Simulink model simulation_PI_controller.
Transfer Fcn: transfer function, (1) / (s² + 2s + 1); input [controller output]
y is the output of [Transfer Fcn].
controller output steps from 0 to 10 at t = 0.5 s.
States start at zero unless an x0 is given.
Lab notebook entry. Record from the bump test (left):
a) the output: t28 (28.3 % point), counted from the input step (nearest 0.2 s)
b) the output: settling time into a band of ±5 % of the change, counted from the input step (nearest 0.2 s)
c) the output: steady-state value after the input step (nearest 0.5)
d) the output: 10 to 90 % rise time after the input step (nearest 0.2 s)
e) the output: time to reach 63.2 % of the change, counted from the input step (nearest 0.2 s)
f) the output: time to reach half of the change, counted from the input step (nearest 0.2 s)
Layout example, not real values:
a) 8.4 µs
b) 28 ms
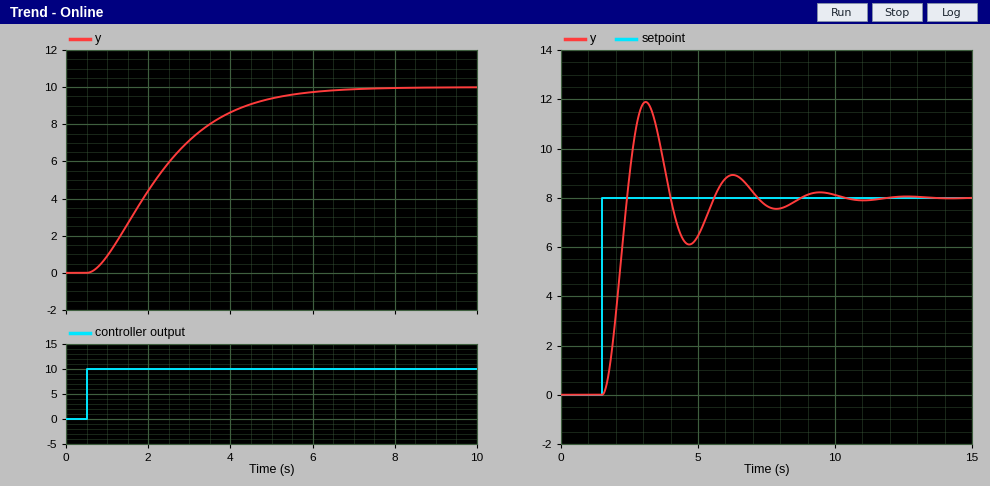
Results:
a) 1.0 s
b) 4.8 s
c) 10.0
d) 3.4 s
e) 2.2 s
f) 1.6 s
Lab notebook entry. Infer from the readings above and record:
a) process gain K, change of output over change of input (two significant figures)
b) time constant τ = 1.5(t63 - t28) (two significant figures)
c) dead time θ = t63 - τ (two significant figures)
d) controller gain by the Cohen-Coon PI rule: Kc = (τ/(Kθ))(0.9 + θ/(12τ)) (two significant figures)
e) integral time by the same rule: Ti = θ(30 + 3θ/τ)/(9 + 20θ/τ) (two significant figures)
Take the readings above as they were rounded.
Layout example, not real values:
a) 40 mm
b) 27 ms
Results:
a) 1.0
b) 1.8 s
c) 0.40 s
d) 4.1
e) 0.91 s
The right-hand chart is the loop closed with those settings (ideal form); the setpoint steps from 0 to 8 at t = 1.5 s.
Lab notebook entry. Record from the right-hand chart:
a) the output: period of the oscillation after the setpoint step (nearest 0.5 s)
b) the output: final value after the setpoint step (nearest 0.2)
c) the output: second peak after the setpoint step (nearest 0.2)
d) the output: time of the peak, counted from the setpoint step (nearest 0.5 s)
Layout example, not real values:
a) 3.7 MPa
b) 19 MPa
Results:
a) 3.0 s
b) 8.0
c) 9.0
d) 1.5 s
